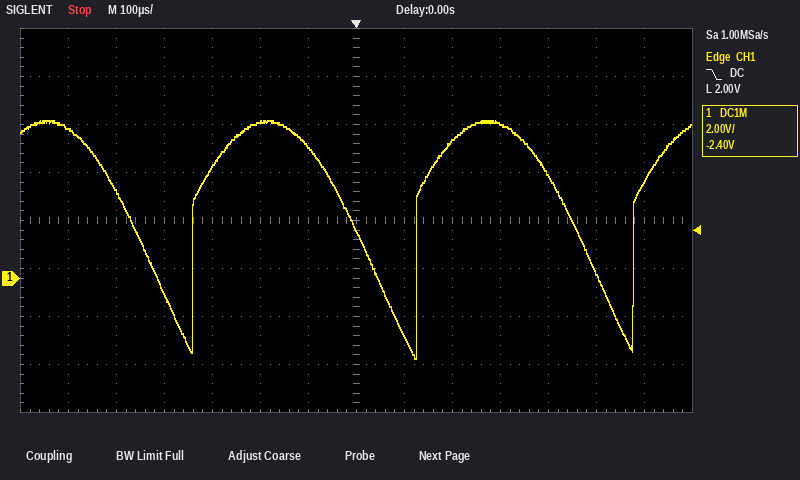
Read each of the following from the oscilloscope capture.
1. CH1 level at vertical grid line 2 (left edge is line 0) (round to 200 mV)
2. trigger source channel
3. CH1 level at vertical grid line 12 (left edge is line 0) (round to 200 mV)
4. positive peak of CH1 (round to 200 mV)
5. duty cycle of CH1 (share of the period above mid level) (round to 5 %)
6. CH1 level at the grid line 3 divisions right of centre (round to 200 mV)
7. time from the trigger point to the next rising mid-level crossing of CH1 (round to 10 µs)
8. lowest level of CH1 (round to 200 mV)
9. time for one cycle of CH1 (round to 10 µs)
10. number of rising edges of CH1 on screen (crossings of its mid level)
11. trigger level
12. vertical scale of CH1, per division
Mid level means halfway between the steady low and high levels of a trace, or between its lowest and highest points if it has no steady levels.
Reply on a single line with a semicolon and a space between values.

3.6 V; CH1; 200 mV; 6.6 V; 75 %; 6.4 V; 130 µs; -3.4 V; 460 µs; 3; 2.00 V; 2 V
